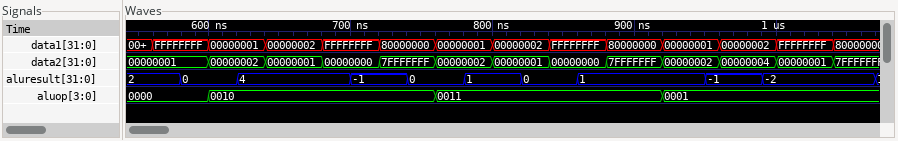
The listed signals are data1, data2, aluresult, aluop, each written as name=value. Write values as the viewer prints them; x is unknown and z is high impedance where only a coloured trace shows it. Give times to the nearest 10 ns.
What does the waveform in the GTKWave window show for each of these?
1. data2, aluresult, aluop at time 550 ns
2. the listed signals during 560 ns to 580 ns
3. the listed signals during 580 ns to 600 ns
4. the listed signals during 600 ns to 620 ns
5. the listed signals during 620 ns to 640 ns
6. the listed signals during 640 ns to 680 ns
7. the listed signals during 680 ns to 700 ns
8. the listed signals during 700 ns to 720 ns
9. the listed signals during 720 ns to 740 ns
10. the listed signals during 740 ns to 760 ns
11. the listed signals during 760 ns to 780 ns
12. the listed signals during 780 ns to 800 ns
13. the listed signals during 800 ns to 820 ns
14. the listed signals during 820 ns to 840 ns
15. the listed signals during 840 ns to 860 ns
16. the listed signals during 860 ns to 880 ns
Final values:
data2=00000001, aluresult=2, aluop=0000
data1=FFFFFFFF, data2=00000001, aluresult=2, aluop=0000
data1=FFFFFFFF, data2=00000001, aluresult=0, aluop=0000
data1=00000001, data2=00000002, aluresult=0, aluop=0010
data1=00000001, data2=00000002, aluresult=4, aluop=0010
data1=00000002, data2=00000001, aluresult=4, aluop=0010
data1=FFFFFFFF, data2=00000000, aluresult=4, aluop=0010
data1=FFFFFFFF, data2=00000000, aluresult=-1, aluop=0010
data1=80000000, data2=7FFFFFFF, aluresult=-1, aluop=0010
data1=80000000, data2=7FFFFFFF, aluresult=0, aluop=0010
data1=00000001, data2=00000002, aluresult=0, aluop=0011
data1=00000001, data2=00000002, aluresult=1, aluop=0011
data1=00000002, data2=00000001, aluresult=1, aluop=0011
data1=00000002, data2=00000001, aluresult=0, aluop=0011
data1=FFFFFFFF, data2=00000000, aluresult=0, aluop=0011
data1=FFFFFFFF, data2=00000000, aluresult=1, aluop=0011
